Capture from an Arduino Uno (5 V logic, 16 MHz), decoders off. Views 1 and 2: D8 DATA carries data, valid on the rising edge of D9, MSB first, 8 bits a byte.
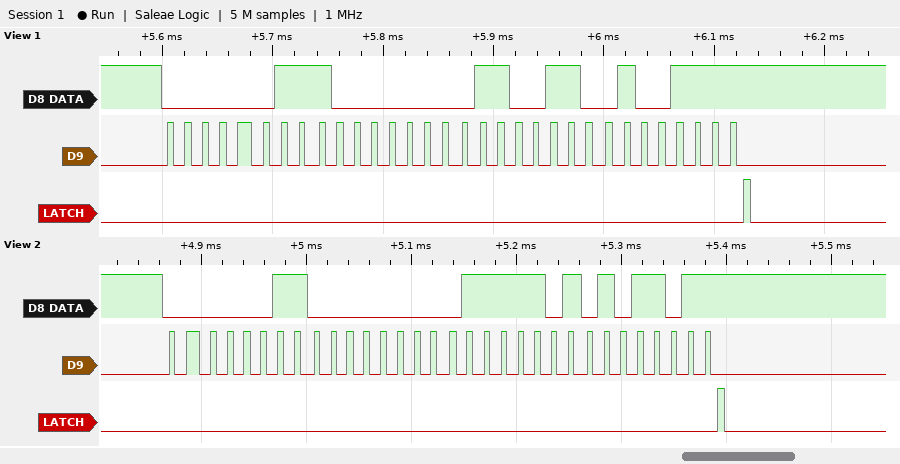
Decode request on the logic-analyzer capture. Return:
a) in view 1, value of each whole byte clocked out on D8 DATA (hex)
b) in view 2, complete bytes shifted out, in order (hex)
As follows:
0x03 0x80 0x66 0x4F
03 00 7D 5B
